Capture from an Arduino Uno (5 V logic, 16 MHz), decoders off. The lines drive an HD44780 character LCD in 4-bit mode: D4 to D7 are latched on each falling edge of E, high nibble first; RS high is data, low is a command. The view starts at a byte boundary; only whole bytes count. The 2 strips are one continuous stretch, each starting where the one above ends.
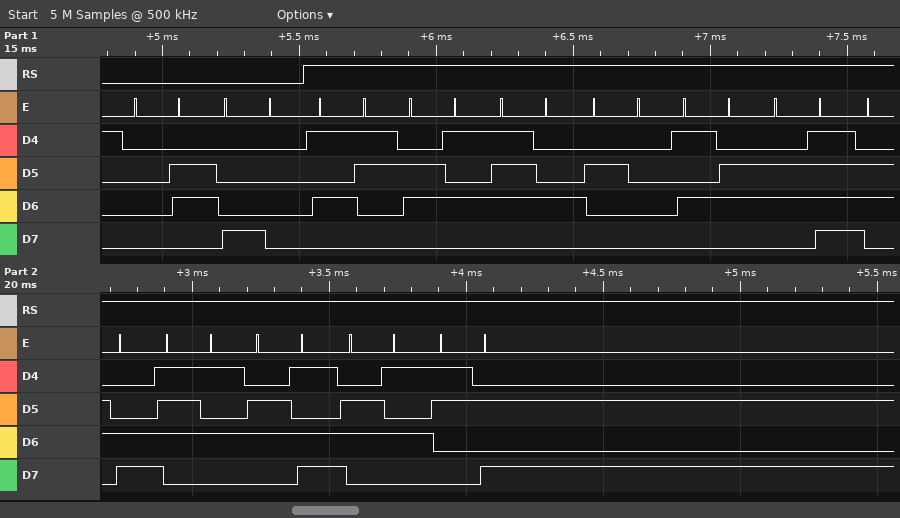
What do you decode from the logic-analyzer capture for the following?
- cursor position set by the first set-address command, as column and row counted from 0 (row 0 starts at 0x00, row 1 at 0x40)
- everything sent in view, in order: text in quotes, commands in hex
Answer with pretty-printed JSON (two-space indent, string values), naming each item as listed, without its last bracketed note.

{
  "cursor position set by the first set-address command, as column and row counted from 0": "column 0, row 0",
  "everything sent in view, in order: text in quotes, commands in hex": "0x06 0x80 \"Set Volume:\""
}
